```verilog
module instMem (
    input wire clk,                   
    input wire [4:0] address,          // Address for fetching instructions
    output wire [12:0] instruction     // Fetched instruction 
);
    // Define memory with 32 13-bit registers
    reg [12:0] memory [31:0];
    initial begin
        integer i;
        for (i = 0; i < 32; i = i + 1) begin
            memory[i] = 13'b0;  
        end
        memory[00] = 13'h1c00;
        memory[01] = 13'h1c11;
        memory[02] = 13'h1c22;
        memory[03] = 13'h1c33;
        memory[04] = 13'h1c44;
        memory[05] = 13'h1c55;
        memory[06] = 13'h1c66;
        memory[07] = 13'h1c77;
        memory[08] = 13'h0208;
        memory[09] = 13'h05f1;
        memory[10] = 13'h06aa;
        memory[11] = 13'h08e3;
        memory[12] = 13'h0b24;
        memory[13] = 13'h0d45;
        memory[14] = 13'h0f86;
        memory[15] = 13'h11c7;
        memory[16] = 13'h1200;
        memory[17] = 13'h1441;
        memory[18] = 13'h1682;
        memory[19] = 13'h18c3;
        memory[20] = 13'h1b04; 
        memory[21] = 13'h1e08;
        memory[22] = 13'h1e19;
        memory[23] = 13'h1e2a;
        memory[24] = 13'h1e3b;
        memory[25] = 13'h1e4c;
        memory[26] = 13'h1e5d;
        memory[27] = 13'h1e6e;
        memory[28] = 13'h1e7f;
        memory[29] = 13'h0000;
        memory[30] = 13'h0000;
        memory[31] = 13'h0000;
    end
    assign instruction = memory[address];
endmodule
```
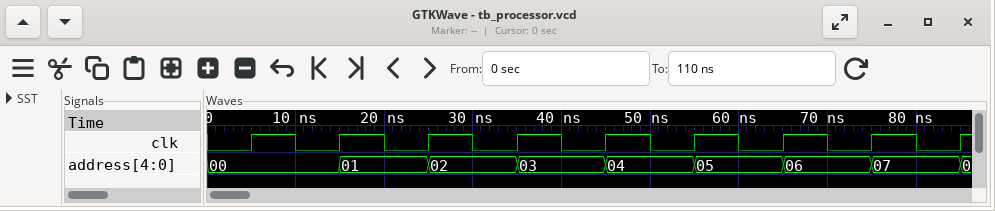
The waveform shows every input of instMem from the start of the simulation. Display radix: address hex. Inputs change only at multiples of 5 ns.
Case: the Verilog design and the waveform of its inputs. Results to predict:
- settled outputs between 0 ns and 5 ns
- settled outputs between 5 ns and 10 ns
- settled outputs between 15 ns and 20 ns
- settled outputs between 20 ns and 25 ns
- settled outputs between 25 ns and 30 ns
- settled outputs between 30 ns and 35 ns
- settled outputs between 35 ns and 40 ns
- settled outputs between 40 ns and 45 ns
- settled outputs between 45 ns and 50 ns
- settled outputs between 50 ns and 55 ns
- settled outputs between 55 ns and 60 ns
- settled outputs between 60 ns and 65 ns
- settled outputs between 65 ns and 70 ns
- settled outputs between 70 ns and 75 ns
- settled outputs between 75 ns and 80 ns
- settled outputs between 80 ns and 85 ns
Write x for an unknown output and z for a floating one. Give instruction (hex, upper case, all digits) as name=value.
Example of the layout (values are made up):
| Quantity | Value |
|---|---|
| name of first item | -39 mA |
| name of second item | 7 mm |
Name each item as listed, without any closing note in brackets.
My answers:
| Quantity | Value |
|---|---|
| settled outputs between 0 ns and 5 ns | instruction=1C00 |
| settled outputs between 5 ns and 10 ns | instruction=1C00 |
| settled outputs between 15 ns and 20 ns | instruction=1C11 |
| settled outputs between 20 ns and 25 ns | instruction=1C11 |
| settled outputs between 25 ns and 30 ns | instruction=1C22 |
| settled outputs between 30 ns and 35 ns | instruction=1C22 |
| settled outputs between 35 ns and 40 ns | instruction=1C33 |
| settled outputs between 40 ns and 45 ns | instruction=1C33 |
| settled outputs between 45 ns and 50 ns | instruction=1C44 |
| settled outputs between 50 ns and 55 ns | instruction=1C44 |
| settled outputs between 55 ns and 60 ns | instruction=1C55 |
| settled outputs between 60 ns and 65 ns | instruction=1C55 |
| settled outputs between 65 ns and 70 ns | instruction=1C66 |
| settled outputs between 70 ns and 75 ns | instruction=1C66 |
| settled outputs between 75 ns and 80 ns | instruction=1C77 |
| settled outputs between 80 ns and 85 ns | instruction=1C77 |
